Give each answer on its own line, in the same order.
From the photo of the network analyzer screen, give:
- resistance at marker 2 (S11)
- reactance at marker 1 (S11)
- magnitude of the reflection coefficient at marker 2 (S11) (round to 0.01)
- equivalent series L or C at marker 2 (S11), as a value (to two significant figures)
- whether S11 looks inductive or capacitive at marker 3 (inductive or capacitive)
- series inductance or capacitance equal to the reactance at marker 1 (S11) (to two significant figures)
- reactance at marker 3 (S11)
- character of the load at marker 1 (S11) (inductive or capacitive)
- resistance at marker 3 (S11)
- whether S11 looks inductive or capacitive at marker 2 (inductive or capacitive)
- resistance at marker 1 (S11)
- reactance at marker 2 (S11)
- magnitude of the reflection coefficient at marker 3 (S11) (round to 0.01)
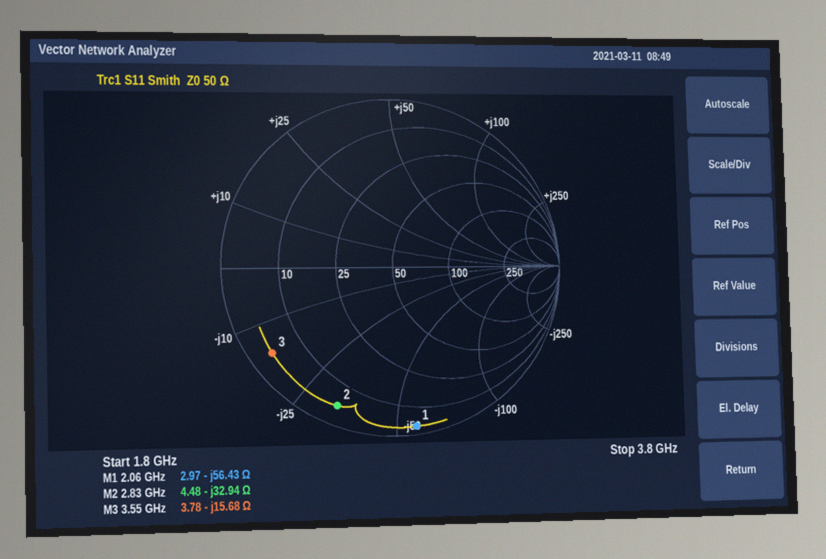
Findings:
4.48 Ω
-56.43 Ω
0.88
1.7 pF
capacitive
1.4 pF
-15.68 Ω
capacitive
3.78 Ω
capacitive
2.97 Ω
-32.94 Ω
0.87
